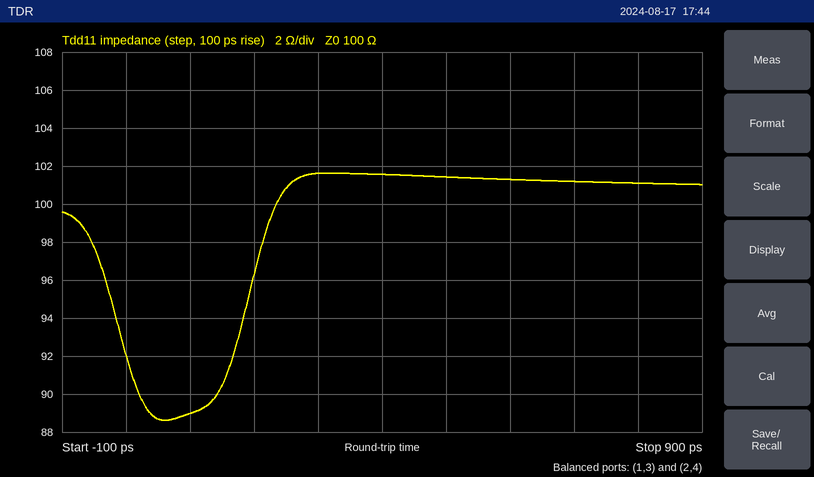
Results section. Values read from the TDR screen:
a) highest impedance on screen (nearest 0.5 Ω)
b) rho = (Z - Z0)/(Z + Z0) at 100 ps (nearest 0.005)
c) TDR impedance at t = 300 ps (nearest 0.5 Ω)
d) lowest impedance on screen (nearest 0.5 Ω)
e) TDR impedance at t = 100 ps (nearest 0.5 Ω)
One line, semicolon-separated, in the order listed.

101.5 Ω; -0.060; 101.5 Ω; 88.5 Ω; 89.0 Ω
